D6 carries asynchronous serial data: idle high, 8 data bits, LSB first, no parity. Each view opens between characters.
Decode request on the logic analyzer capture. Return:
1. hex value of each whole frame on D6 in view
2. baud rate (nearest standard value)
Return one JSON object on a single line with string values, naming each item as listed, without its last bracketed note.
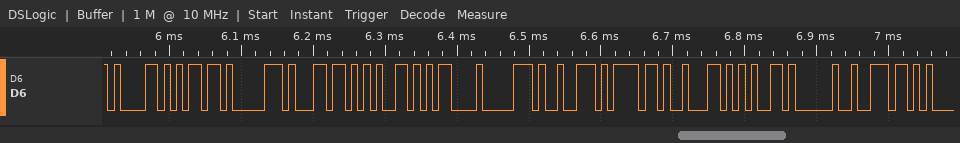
{"hex value of each whole frame on D6 in view": "61, 6D, 70, 6C, 65, 0D, 70, 72, 6F, 62, 65, 20, 6E", "baud rate": "115200 baud"}
